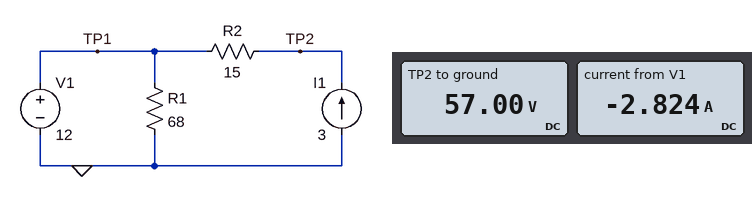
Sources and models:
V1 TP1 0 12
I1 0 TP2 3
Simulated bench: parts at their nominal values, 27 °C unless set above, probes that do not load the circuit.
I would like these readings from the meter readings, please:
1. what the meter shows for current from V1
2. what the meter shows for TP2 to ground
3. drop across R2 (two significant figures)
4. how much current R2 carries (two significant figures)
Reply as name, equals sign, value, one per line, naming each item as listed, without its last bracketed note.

what the meter shows for current from V1 = -2.824 A
what the meter shows for TP2 to ground = 57.00 V
drop across R2 = 45 V
how much current R2 carries = 3.0 A
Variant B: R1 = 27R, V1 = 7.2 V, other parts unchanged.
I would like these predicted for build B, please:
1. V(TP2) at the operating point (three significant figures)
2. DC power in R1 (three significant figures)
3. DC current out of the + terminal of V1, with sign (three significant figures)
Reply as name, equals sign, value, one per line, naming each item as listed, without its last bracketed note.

V(TP2) at the operating point = 52.2 V
DC power in R1 = 1.92 W
DC current out of the + terminal of V1, with sign = -2.73 A
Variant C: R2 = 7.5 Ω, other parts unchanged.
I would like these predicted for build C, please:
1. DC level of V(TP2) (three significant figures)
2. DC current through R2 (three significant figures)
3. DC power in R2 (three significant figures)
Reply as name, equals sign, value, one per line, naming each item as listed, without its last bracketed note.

DC level of V(TP2) = 34.5 V
DC current through R2 = 3.00 A
DC power in R2 = 67.5 W
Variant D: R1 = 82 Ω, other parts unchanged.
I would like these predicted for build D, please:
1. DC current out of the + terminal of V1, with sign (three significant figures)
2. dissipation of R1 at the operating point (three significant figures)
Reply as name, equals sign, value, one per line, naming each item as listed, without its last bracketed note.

DC current out of the + terminal of V1, with sign = -2.85 A
dissipation of R1 at the operating point = 1.76 W
